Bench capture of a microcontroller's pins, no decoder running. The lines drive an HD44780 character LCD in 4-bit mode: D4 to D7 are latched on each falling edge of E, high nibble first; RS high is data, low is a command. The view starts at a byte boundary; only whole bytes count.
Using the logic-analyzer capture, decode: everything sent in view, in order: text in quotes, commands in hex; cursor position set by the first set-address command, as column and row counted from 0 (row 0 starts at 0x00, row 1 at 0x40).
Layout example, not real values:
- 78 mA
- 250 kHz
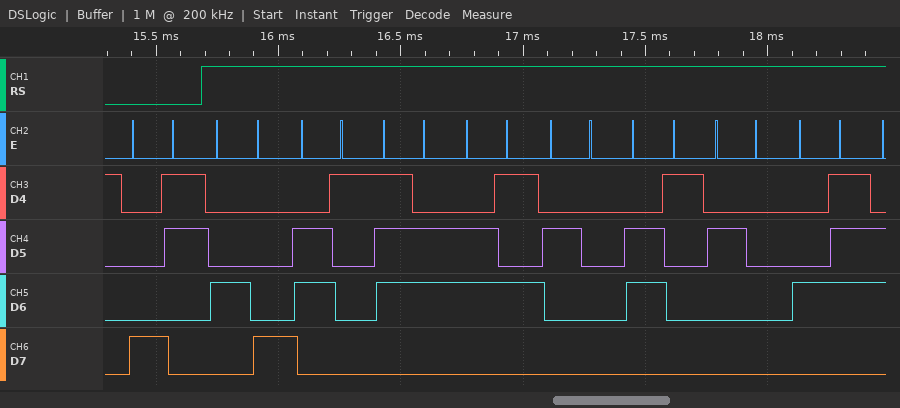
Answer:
- 0x83 "Have a G"
- column 3, row 0
